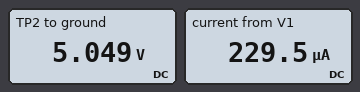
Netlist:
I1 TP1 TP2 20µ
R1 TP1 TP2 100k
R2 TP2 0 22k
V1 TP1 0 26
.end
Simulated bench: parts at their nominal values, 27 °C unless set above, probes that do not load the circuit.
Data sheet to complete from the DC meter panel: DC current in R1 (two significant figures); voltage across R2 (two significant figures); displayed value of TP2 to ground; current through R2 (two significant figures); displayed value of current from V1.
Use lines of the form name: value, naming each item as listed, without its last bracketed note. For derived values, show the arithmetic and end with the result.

DC current in R1: (26 V - 5.049 V) / 100 kΩ = 210 µA
voltage across R2: 5.049 V = 5.0 V
displayed value of TP2 to ground: 5.049 V
current through R2: (5.049 V) / 22 kΩ = 230 µA
displayed value of current from V1: 229.5 µA
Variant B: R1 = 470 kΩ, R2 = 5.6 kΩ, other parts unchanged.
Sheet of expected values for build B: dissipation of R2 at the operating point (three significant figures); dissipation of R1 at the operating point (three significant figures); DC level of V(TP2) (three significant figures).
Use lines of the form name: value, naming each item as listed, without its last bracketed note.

dissipation of R2 at the operating point: 31.0 µW
dissipation of R1 at the operating point: 1.39 mW
DC level of V(TP2): 417 mV
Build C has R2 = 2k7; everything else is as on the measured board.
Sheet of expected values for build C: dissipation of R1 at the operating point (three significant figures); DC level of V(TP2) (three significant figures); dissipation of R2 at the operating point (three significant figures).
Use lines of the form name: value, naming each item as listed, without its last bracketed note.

dissipation of R1 at the operating point: 6.38 mW
DC level of V(TP2): 736 mV
dissipation of R2 at the operating point: 201 µW
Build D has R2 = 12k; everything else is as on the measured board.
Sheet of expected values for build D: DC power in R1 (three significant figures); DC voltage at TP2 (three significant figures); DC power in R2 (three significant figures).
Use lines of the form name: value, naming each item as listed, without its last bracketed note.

DC power in R1: 5.29 mW
DC voltage at TP2: 3.00 V
DC power in R2: 750 µW
